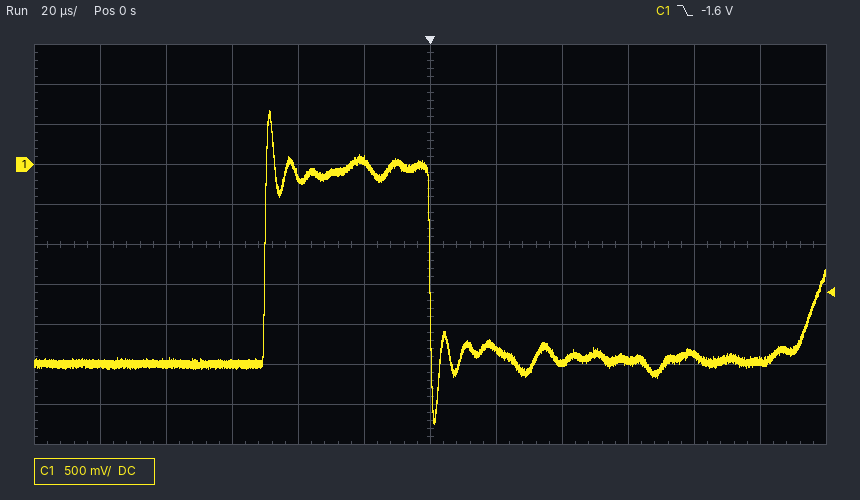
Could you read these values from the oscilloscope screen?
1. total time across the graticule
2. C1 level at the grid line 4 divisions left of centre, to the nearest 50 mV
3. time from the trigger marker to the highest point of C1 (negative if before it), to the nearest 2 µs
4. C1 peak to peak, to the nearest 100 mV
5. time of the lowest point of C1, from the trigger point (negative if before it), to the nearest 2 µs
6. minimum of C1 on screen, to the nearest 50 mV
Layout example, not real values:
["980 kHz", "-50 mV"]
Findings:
["240 µs", "-2.50 V", "-48 µs", "3.90 V", "+2 µs", "-3.25 V"]
